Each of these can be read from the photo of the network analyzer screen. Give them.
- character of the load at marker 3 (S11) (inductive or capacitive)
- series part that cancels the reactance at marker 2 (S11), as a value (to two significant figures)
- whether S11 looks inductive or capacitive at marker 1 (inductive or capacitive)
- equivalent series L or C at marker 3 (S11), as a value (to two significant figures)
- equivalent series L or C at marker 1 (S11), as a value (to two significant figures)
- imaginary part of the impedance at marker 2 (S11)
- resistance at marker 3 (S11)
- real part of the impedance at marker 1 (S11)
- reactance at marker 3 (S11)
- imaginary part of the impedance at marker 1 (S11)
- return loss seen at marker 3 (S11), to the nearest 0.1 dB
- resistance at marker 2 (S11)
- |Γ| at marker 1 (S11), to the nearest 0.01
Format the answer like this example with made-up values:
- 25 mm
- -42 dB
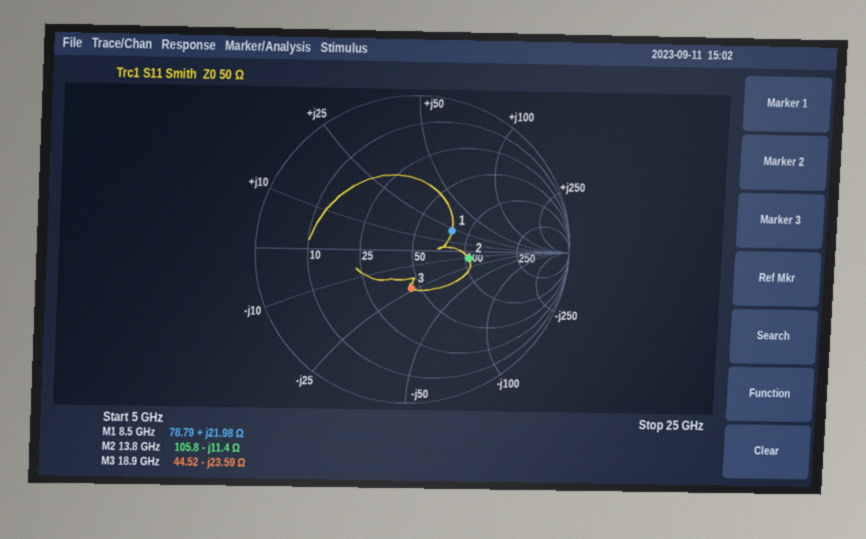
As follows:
- capacitive
- 130 pH
- inductive
- 360 fF
- 410 pH
- -11.4 Ω
- 44.52 Ω
- 78.79 Ω
- -23.59 Ω
- +21.98 Ω
- 12.1 dB
- 105.8 Ω
- 0.28
